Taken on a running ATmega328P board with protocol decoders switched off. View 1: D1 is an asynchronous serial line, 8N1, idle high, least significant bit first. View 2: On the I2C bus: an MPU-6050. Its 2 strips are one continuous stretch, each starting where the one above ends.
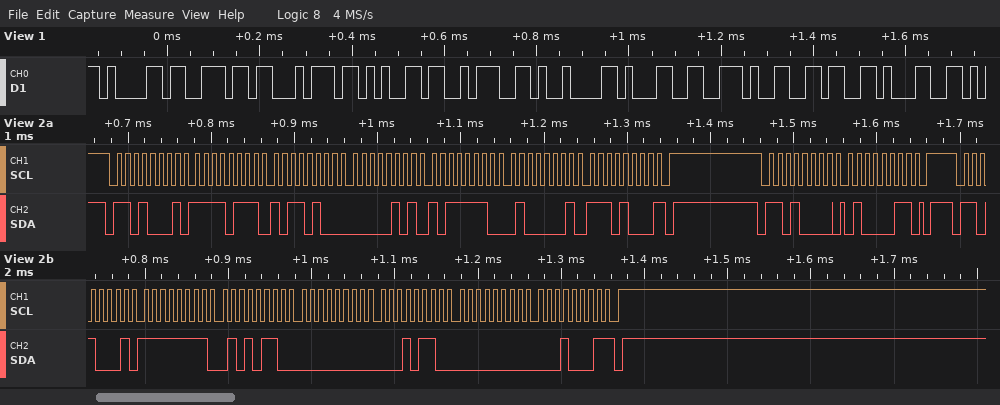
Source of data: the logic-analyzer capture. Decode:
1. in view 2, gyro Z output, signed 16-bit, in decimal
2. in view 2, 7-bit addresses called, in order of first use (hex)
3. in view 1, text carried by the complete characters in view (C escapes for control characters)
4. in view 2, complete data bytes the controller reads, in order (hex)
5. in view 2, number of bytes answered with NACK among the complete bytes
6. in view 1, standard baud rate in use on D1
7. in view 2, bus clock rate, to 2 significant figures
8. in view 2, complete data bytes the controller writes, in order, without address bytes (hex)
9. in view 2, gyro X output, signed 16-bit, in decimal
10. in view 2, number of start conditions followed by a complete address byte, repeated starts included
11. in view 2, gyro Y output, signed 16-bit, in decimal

17
0x68
"ante:\t1.61"
F7 B4 05 BE 41 E8 FF 56 00 16 00 11
2
57600 baud
100 kHz
43
-170
3
22
